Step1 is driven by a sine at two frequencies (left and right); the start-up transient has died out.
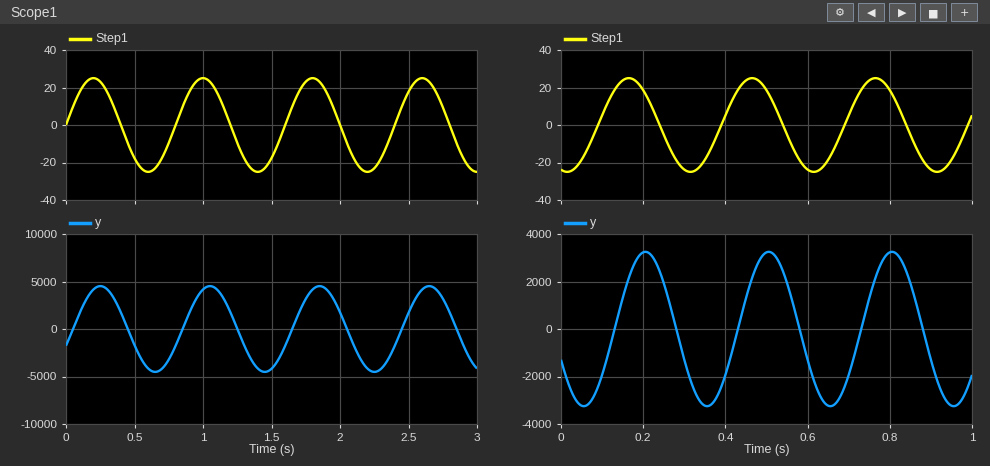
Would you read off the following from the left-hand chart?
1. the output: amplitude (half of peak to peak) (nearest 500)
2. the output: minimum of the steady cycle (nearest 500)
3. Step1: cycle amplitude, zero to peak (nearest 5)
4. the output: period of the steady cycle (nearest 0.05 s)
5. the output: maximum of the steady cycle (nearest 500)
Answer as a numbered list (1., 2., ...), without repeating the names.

1. 4500
2. -4500
3. 25
4. 0.80 s
5. 4500
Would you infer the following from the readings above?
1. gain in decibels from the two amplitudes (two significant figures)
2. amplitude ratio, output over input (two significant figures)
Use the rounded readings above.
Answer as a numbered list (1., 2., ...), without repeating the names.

1. 45 dB
2. 180
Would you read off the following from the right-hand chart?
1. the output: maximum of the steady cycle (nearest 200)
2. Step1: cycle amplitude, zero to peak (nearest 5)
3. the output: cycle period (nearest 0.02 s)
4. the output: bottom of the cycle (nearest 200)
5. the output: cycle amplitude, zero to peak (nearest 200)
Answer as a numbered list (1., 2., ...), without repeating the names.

1. 3200
2. 25
3. 0.30 s
4. -3200
5. 3200
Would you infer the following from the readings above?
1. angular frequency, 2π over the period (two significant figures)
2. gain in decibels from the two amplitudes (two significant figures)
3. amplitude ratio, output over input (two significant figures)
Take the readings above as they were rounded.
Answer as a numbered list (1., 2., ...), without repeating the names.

1. 21 rad/s
2. 42 dB
3. 130
